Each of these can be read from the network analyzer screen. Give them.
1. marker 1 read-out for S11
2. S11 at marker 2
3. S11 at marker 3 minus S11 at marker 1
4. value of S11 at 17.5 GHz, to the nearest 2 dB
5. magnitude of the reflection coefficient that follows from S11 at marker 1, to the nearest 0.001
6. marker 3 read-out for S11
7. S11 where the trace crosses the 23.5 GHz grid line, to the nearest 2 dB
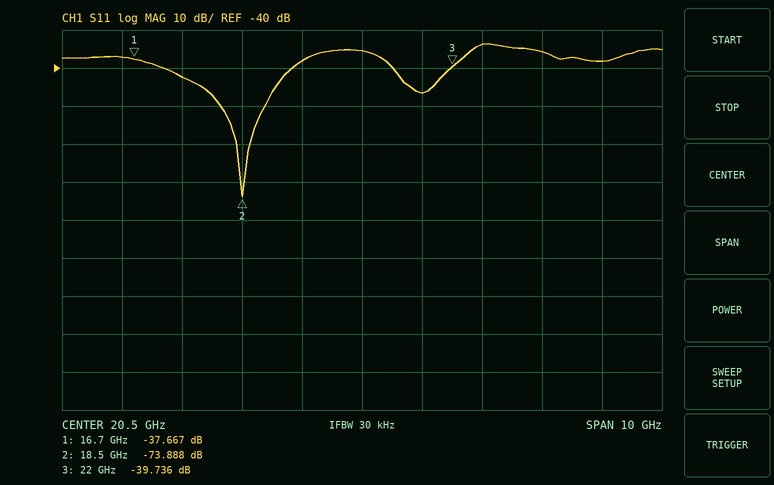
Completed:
-37.667 dB
-73.888 dB
-2.069 dB
-42 dB
0.013
-39.736 dB
-36 dB
